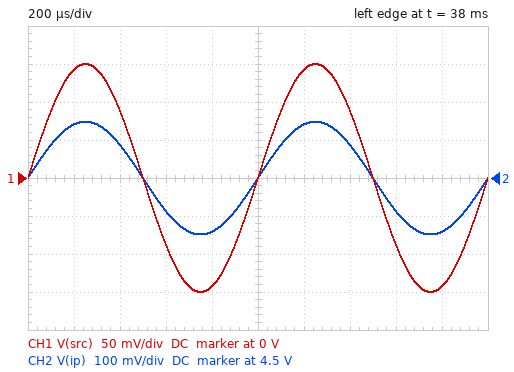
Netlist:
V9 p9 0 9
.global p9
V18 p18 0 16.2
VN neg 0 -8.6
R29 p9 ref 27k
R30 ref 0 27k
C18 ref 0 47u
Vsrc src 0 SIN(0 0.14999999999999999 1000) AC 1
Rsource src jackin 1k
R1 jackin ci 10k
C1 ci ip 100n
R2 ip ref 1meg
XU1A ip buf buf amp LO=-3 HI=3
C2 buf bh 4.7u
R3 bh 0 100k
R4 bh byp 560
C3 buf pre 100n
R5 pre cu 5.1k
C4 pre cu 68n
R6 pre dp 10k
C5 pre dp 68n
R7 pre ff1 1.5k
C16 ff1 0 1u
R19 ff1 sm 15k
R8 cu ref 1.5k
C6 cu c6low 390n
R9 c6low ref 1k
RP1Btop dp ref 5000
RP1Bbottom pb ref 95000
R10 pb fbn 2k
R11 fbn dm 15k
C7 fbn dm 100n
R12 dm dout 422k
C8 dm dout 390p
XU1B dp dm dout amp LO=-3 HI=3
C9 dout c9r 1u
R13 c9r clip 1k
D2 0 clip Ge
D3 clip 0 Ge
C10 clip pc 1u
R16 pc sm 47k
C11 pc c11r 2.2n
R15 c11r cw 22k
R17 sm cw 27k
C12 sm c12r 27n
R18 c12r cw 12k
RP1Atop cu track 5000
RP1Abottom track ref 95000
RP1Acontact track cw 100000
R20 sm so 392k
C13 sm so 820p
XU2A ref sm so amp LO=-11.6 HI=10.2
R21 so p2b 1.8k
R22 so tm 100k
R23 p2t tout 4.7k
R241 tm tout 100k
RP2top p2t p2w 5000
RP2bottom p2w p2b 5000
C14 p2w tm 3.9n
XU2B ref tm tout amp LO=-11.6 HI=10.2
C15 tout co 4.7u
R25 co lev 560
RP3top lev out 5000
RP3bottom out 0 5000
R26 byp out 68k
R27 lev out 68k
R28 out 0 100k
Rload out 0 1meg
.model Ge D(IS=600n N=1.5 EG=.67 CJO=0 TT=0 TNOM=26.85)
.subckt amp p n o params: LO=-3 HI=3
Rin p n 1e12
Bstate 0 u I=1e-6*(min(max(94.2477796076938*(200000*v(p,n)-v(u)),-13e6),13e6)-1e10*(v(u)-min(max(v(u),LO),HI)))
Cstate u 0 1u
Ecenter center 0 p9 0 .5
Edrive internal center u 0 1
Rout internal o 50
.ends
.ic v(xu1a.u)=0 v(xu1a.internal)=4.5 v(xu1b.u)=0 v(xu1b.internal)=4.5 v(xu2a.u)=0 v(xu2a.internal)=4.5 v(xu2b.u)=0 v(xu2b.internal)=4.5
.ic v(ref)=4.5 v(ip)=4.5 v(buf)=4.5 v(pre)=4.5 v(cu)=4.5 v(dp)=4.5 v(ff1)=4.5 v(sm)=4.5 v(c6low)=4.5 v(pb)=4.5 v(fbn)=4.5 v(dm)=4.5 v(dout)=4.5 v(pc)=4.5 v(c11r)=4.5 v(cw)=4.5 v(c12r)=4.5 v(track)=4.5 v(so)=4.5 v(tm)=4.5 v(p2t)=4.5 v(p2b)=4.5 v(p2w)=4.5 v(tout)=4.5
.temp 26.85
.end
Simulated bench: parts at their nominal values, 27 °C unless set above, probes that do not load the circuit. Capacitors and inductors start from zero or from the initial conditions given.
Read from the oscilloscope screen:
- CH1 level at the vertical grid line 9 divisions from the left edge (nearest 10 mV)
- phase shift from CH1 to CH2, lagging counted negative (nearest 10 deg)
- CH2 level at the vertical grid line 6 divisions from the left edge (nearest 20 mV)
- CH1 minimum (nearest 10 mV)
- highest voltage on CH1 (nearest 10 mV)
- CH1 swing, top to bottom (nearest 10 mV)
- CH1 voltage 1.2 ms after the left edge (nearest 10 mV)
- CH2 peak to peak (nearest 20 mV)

-140 mV
0 deg
4.64 V
-150 mV
150 mV
300 mV
140 mV
300 mV
